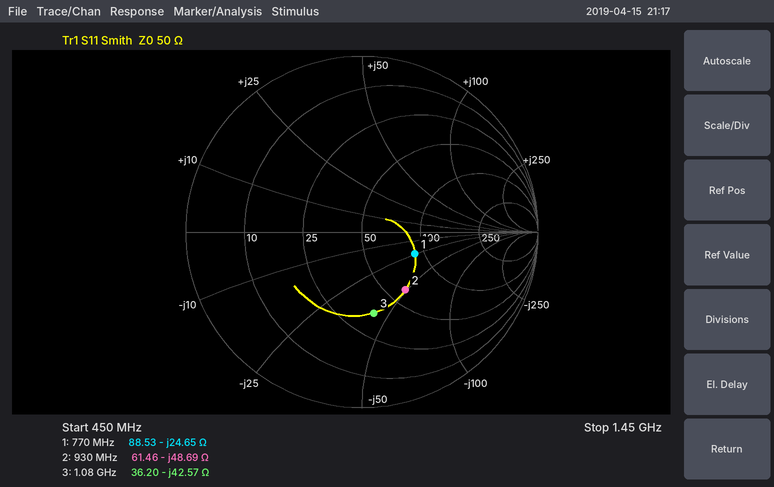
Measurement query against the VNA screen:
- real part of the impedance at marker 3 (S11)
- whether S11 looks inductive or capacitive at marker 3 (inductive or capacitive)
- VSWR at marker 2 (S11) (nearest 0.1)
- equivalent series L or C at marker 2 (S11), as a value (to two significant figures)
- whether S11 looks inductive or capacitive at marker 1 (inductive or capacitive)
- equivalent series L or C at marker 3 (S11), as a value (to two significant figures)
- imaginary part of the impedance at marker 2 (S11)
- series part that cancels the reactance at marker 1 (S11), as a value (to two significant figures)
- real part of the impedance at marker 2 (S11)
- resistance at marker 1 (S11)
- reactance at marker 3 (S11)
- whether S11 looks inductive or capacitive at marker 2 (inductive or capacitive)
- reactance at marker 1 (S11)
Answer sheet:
36.20 Ω
capacitive
2.4
3.5 pF
capacitive
3.5 pF
-48.69 Ω
5.1 nH
61.46 Ω
88.53 Ω
-42.57 Ω
capacitive
-24.65 Ω
